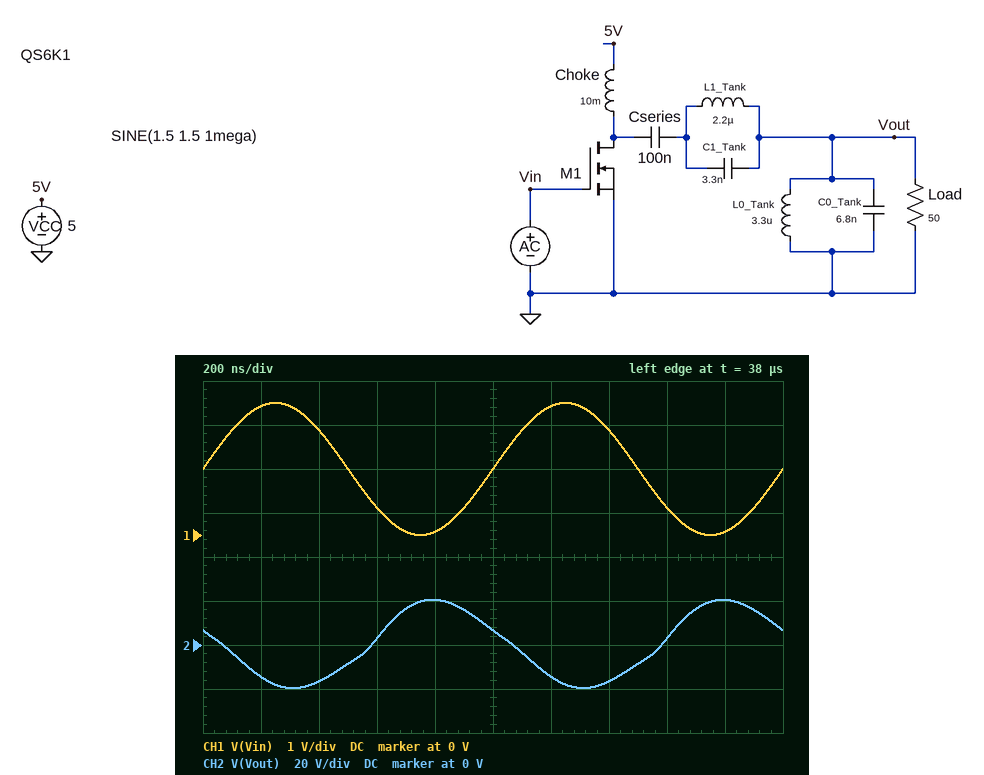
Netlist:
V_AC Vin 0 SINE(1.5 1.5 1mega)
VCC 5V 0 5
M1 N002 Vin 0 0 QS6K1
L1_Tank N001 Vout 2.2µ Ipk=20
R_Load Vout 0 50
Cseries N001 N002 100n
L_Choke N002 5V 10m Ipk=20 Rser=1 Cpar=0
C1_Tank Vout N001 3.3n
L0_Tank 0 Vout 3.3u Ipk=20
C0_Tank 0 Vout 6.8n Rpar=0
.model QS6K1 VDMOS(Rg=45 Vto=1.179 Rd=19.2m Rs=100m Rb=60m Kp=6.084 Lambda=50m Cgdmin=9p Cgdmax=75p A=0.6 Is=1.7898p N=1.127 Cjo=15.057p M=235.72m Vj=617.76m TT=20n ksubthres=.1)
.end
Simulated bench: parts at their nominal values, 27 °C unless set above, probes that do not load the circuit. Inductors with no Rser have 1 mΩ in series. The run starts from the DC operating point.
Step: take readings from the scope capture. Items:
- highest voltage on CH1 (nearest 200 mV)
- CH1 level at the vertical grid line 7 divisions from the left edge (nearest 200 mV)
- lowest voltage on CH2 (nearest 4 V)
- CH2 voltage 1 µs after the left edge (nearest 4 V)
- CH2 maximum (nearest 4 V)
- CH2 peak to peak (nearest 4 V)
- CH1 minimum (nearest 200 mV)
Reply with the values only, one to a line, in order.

3.0 V
2.4 V
-20 V
8 V
20 V
40 V
0 V
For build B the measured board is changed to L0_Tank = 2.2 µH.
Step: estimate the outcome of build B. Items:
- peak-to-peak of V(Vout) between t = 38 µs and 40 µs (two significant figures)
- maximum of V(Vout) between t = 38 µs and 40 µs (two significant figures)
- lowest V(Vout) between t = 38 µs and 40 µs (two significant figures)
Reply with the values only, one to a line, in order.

46 V
25 V
-21 V
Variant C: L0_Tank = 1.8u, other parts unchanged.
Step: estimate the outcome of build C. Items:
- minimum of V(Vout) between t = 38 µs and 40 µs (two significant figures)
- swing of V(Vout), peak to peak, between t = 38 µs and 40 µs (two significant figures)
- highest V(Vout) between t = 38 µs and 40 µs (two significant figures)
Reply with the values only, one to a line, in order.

-21 V
47 V
26 V
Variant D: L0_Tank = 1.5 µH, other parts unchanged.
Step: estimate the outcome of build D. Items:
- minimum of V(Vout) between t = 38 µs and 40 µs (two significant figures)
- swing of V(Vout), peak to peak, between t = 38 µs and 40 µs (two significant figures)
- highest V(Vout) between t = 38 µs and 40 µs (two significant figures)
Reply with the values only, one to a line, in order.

-19 V
46 V
27 V
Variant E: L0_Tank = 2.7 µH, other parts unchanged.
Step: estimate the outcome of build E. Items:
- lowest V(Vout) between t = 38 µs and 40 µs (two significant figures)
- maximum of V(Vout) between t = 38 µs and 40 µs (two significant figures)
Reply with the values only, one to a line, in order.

-21 V
23 V
